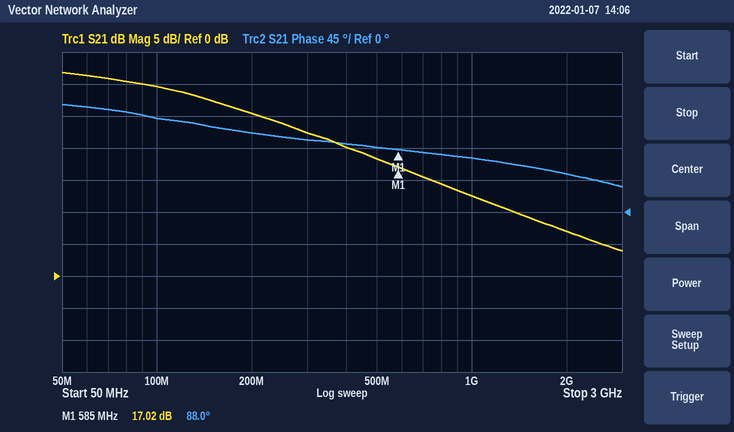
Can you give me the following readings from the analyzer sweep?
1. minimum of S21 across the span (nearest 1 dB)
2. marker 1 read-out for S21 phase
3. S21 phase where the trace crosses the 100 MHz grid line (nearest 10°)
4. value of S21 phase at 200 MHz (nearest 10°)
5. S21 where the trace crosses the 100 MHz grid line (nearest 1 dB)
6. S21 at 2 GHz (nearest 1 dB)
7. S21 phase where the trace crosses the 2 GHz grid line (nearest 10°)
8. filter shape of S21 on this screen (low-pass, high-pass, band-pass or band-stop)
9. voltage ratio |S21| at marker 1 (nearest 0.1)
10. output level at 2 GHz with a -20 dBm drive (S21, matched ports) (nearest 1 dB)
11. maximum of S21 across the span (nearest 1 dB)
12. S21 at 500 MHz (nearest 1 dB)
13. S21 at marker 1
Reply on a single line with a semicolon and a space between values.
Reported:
4 dB; 88.0°; 130°; 110°; 30 dB; 7 dB; 50°; low-pass; 7.1; -13 dBm; 32 dB; 18 dB; 17.02 dB
